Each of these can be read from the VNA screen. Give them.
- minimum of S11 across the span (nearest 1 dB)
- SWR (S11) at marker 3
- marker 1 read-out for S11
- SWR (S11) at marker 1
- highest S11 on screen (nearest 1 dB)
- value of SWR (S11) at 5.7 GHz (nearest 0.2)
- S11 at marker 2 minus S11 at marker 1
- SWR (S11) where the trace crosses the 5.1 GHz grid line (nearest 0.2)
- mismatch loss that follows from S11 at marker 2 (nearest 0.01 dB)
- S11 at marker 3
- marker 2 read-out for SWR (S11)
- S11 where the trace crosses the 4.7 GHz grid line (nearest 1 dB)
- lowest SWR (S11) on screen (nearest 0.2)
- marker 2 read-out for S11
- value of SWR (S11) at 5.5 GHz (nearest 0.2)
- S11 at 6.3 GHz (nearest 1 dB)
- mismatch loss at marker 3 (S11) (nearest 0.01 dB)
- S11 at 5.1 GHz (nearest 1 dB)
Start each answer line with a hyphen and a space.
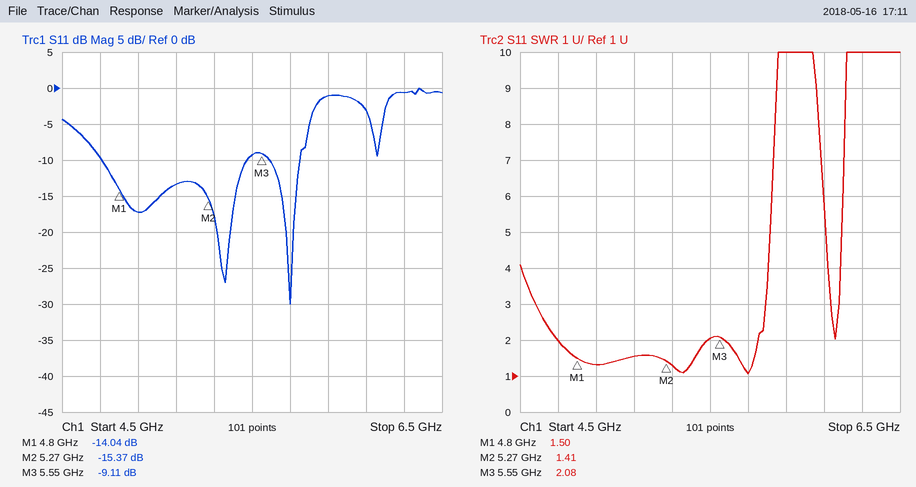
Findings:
- -30 dB
- 2.08
- -14.04 dB
- 1.50
- 0 dB
- 1.0
- -1.33 dB
- 1.6
- 0.13 dB
- -9.11 dB
- 1.41
- -10 dB
- 1.0
- -15.37 dB
- 2.0
- -1 dB
- 0.57 dB
- -13 dB
